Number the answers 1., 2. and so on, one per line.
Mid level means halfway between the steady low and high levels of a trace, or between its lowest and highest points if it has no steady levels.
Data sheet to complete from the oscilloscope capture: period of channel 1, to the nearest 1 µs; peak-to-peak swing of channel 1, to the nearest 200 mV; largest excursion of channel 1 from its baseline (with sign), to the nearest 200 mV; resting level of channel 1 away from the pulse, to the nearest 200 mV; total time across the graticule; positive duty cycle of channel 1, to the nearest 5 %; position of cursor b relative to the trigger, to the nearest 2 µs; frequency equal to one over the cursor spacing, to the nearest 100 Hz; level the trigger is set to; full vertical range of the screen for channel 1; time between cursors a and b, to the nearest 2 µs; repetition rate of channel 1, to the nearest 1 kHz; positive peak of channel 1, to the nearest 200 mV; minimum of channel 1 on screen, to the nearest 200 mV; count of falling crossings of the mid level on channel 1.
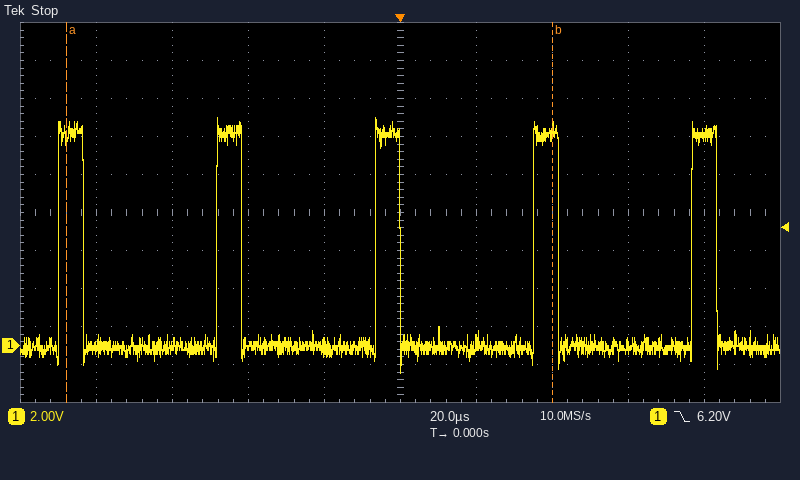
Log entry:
1. 42 µs
2. 13.4 V
3. +12.0 V
4. 0.0 V
5. 200 µs
6. 15 %
7. +40 µs
8. 7.8 kHz
9. 6.20 V
10. 20 V
11. 128 µs
12. 24 kHz
13. 12.0 V
14. -1.4 V
15. 5
